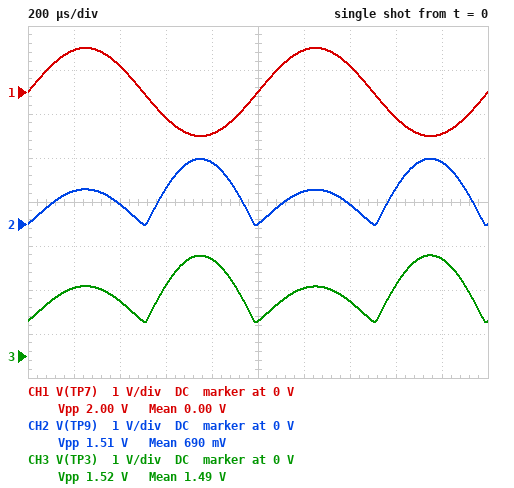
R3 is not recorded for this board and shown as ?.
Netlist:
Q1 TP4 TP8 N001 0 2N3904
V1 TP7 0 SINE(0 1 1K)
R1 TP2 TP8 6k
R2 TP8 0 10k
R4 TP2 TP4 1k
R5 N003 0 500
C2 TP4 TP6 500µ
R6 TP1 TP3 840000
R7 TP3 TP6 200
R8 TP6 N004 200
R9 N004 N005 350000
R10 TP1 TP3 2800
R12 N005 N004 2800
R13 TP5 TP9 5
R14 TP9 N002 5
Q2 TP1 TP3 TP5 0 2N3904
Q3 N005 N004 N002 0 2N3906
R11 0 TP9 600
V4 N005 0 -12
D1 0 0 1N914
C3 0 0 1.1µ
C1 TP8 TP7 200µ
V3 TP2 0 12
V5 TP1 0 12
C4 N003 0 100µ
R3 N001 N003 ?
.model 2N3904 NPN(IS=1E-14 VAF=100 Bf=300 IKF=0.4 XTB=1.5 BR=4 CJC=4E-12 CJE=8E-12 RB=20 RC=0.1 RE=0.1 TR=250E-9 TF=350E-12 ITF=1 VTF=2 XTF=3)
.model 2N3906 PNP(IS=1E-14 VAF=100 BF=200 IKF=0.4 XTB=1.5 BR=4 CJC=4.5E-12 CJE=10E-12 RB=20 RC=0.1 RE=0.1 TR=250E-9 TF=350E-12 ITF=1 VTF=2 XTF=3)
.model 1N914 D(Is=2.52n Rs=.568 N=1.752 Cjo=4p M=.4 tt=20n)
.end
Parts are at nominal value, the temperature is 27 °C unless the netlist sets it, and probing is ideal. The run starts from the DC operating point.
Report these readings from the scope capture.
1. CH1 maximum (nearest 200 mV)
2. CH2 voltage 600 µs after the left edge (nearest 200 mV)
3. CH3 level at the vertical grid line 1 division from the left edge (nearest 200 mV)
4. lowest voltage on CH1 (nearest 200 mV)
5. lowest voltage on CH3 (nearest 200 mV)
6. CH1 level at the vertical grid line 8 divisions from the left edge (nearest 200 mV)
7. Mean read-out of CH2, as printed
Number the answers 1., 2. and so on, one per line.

1. 1.0 V
2. 800 mV
3. 1.6 V
4. -1.0 V
5. 800 mV
6. -600 mV
7. 690 mV
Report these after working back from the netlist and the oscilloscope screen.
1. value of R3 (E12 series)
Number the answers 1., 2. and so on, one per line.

1. 330 Ω
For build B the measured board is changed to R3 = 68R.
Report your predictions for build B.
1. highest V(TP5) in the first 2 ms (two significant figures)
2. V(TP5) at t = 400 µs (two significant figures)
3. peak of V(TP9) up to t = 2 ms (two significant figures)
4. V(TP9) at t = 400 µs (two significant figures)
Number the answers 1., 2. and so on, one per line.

1. 4.2 V
2. 430 mV
3. 4.1 V
4. 360 mV
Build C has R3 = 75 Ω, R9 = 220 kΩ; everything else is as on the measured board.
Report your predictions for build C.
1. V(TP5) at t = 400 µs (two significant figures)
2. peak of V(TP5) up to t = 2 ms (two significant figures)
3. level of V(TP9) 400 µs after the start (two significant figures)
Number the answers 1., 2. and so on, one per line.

1. 410 mV
2. 4.1 V
3. 340 mV
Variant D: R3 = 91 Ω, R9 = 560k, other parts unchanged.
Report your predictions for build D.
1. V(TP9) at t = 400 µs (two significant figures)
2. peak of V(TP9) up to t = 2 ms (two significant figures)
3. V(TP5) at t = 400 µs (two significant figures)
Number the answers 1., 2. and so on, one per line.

1. 400 mV
2. 4.1 V
3. 470 mV
